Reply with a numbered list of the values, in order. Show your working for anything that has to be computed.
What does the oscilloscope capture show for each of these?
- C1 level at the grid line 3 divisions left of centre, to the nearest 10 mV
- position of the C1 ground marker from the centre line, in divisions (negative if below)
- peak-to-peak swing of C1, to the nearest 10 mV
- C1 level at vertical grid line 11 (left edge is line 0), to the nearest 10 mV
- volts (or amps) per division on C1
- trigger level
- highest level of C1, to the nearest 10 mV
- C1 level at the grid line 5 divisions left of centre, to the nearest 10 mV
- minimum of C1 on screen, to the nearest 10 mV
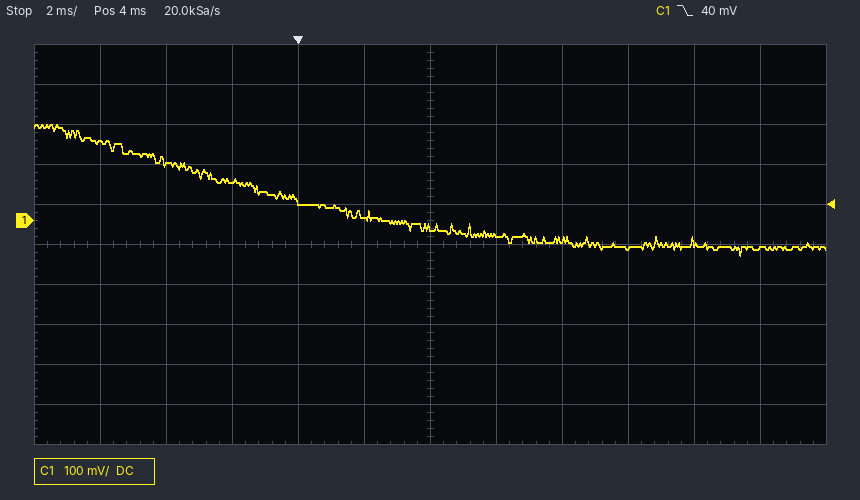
1. 100 mV
2. +0.6 div
3. 240 mV − (-90 mV) = 330 mV
4. -70 mV
5. 100 mV
6. 40 mV
7. 240 mV
8. 200 mV
9. -90 mV
